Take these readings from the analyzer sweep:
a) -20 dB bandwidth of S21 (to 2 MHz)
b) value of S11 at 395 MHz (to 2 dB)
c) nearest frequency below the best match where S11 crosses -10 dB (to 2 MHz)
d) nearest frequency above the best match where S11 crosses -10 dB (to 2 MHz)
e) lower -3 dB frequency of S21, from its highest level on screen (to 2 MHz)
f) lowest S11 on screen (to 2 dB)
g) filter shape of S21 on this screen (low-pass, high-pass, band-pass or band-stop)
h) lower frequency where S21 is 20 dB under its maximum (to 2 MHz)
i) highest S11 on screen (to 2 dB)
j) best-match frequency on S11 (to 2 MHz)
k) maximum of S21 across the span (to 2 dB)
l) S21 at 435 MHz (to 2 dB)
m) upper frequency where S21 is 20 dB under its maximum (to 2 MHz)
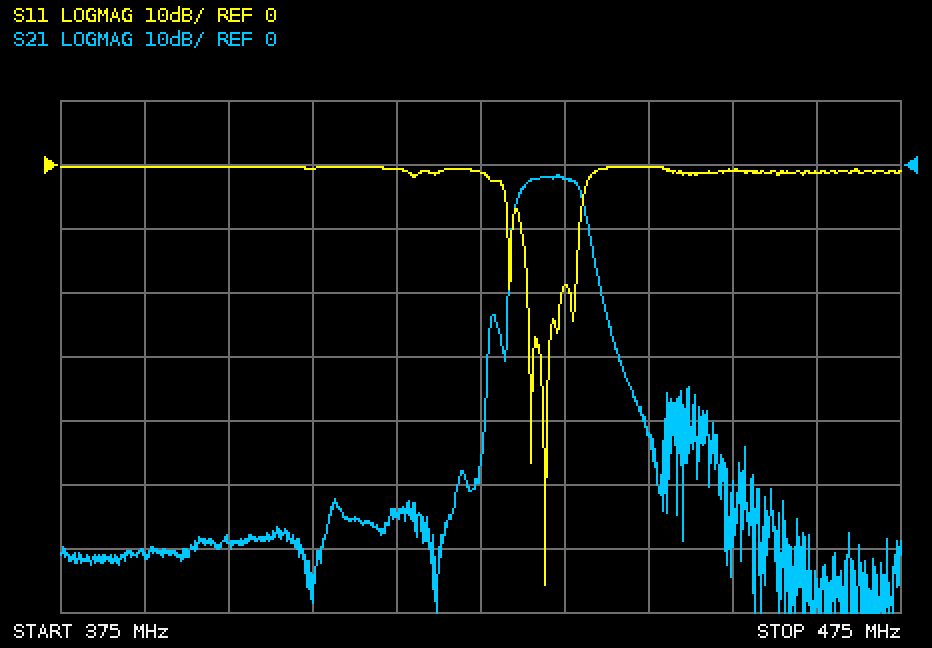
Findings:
12 MHz
0 dB
430 MHz
436 MHz
430 MHz
-66 dB
band-pass
428 MHz
0 dB
432 MHz
-2 dB
-2 dB
440 MHz
